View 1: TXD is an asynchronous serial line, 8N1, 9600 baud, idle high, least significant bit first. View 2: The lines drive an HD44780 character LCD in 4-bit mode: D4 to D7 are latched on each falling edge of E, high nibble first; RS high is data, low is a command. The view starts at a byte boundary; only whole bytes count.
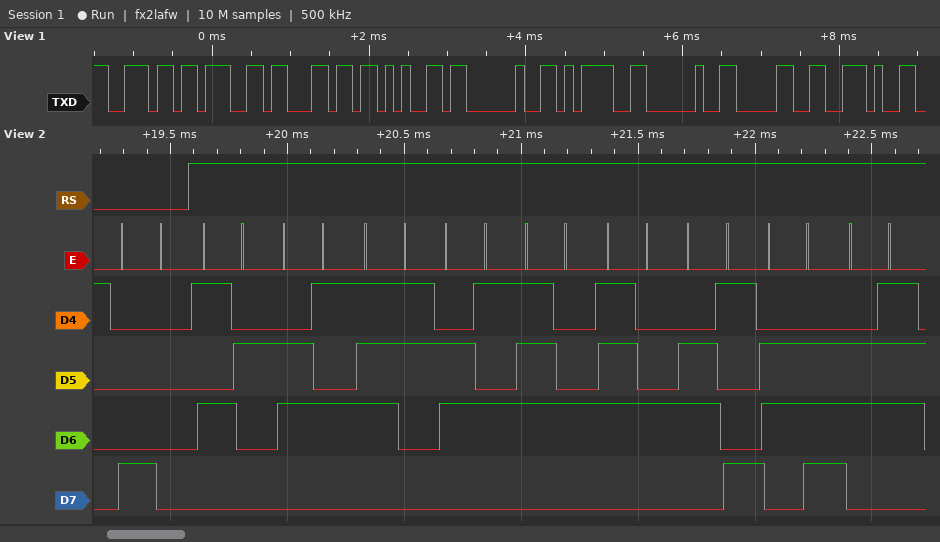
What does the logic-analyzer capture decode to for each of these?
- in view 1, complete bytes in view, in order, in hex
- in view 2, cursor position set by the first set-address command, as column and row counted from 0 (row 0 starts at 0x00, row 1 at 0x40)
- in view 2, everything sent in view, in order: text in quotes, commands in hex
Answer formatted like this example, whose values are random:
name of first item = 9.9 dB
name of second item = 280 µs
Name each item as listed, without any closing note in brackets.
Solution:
in view 1, complete bytes in view, in order, in hex = 6E 67 6C 65 20 3D 20 30 2E
in view 2, cursor position set by the first set-address command, as column and row counted from 0 = column 0, row 0
in view 2, everything sent in view, in order: text in quotes, commands in hex = 0x80 "Resetting"
